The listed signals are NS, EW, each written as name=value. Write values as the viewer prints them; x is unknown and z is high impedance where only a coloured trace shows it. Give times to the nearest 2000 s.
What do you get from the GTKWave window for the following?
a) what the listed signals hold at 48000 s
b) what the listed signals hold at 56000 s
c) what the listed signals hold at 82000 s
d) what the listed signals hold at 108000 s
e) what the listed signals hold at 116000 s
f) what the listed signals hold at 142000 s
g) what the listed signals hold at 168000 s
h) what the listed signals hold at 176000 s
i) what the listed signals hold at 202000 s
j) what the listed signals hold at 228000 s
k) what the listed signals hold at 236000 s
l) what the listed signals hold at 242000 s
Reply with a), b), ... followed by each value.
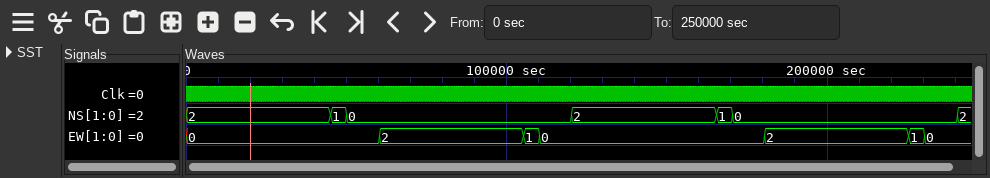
a) NS=1, EW=0
b) NS=0, EW=0
c) NS=0, EW=2
d) NS=0, EW=1
e) NS=0, EW=0
f) NS=2, EW=0
g) NS=1, EW=0
h) NS=0, EW=0
i) NS=0, EW=2
j) NS=0, EW=1
k) NS=0, EW=0
l) NS=2, EW=0
